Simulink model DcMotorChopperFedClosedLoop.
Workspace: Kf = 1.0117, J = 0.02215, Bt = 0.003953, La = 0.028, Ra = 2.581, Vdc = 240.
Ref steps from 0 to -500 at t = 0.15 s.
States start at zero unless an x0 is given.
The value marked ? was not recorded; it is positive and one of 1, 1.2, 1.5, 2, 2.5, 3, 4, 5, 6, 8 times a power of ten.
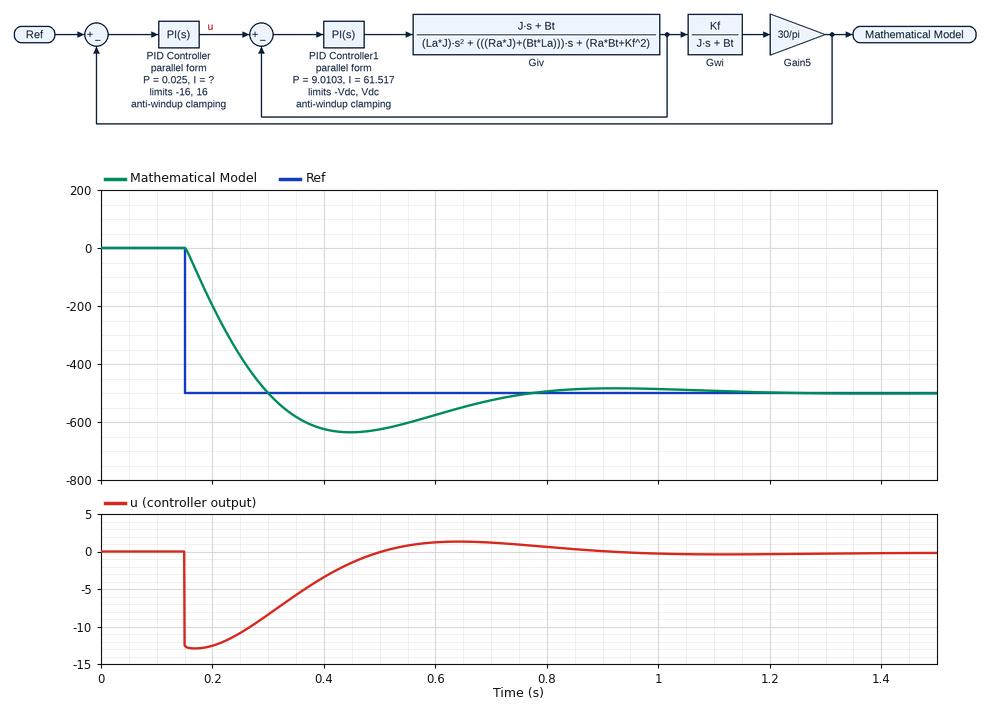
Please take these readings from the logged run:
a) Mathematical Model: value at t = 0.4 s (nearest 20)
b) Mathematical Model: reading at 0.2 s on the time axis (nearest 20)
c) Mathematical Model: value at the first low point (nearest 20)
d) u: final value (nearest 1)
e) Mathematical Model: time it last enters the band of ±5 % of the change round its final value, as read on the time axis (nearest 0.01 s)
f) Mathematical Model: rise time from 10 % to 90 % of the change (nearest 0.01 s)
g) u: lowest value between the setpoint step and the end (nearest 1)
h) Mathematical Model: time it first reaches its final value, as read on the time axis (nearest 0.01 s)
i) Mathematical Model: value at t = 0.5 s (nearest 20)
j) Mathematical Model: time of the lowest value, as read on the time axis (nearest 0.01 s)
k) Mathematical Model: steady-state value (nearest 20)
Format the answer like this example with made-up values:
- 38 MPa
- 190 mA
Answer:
- -620
- -200
- -640
- 0
- 0.70 s
- 0.11 s
- -13
- 0.30 s
- -620
- 0.45 s
- -500
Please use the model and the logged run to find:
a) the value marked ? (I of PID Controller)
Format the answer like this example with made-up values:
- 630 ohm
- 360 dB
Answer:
- 0.25
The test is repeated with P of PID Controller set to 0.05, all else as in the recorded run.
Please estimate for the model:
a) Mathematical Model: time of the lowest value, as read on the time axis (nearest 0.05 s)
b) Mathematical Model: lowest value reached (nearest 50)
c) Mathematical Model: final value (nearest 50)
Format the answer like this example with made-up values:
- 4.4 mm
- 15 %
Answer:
- 0.50 s
- -550
- -500
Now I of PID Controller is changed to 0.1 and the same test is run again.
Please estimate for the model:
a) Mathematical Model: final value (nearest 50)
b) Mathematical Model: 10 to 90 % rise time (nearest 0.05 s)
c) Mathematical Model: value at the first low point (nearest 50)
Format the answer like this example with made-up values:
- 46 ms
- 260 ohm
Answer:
- -500
- 0.15 s
- -600
